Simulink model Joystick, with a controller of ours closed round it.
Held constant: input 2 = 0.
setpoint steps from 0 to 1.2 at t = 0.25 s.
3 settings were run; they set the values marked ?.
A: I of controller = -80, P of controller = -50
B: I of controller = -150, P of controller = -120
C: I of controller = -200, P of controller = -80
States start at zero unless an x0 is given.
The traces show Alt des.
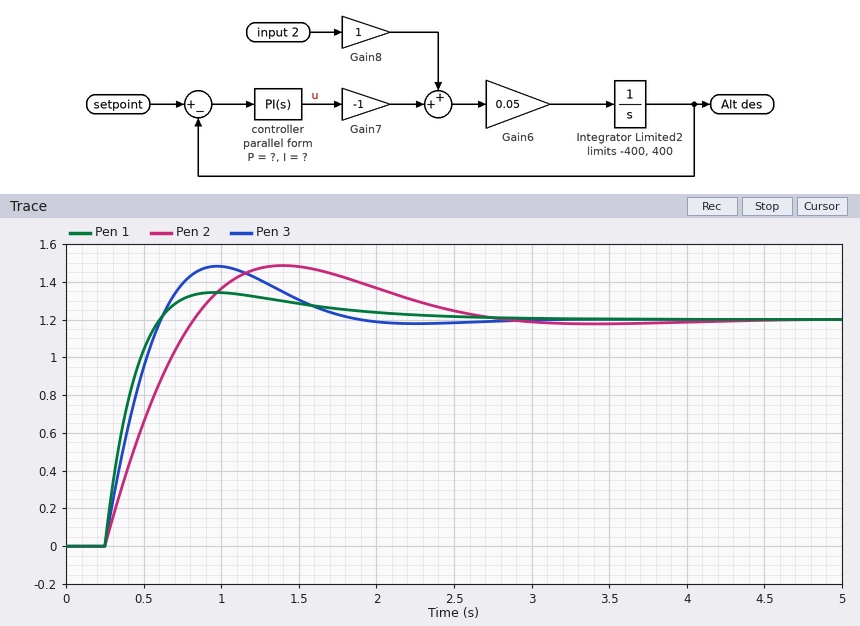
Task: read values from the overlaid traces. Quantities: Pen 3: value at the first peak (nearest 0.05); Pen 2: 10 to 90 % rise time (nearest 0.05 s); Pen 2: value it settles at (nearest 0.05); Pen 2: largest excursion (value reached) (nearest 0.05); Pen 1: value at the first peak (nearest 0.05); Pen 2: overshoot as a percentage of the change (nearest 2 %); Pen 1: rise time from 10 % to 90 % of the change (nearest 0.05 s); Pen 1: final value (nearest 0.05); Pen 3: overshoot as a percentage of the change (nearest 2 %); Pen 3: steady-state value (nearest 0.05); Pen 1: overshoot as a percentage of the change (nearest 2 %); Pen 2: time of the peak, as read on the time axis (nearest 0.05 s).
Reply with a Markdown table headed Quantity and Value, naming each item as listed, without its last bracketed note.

| Quantity | Value |
|---|---|
| Pen 3: value at the first peak | 1.50 |
| Pen 2: 10 to 90 % rise time | 0.45 s |
| Pen 2: value it settles at | 1.20 |
| Pen 2: largest excursion (value reached) | 1.50 |
| Pen 1: value at the first peak | 1.35 |
| Pen 2: overshoot as a percentage of the change | 24 % |
| Pen 1: rise time from 10 % to 90 % of the change | 0.25 s |
| Pen 1: final value | 1.20 |
| Pen 3: overshoot as a percentage of the change | 24 % |
| Pen 3: steady-state value | 1.20 |
| Pen 1: overshoot as a percentage of the change | 12 % |
| Pen 2: time of the peak, as read on the time axis | 1.40 s |
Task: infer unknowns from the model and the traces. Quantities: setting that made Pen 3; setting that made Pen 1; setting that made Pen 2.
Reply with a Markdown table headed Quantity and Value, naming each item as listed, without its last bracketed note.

| Quantity | Value |
|---|---|
| setting that made Pen 3 | C |
| setting that made Pen 1 | B |
| setting that made Pen 2 | A |
